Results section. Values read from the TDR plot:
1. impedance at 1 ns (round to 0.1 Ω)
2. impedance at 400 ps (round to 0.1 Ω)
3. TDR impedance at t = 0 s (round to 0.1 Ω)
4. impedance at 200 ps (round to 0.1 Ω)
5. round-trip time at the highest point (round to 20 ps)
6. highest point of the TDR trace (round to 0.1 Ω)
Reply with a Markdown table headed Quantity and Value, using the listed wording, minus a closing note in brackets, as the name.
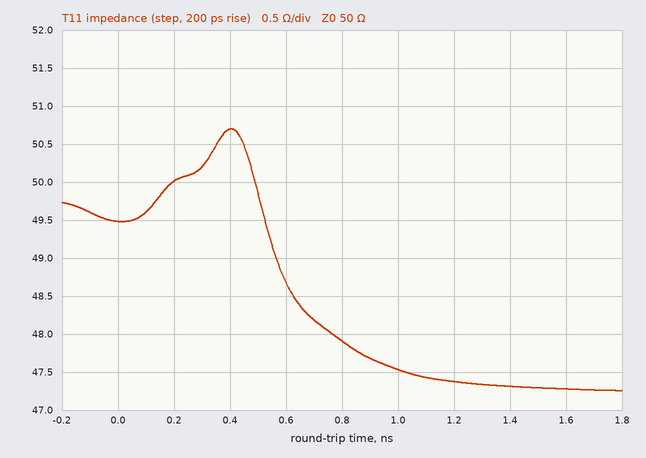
| Quantity | Value |
|---|---|
| impedance at 1 ns | 47.5 Ω |
| impedance at 400 ps | 50.7 Ω |
| TDR impedance at t = 0 s | 49.5 Ω |
| impedance at 200 ps | 50.0 Ω |
| round-trip time at the highest point | 400 ps |
| highest point of the TDR trace | 50.7 Ω |
